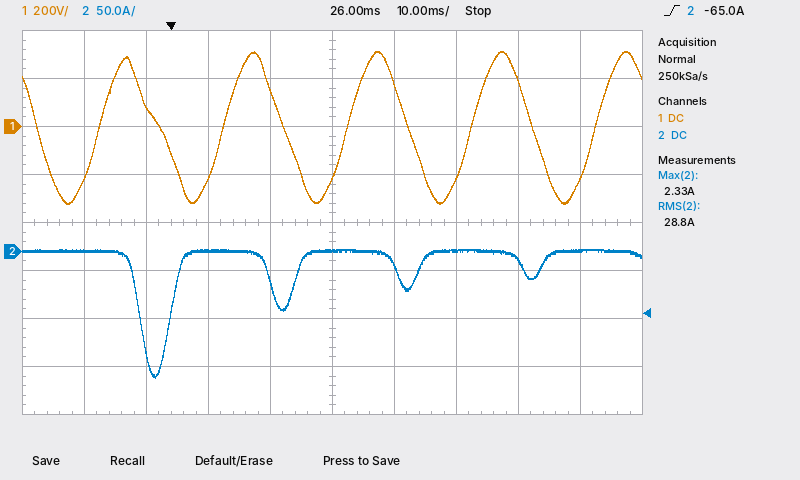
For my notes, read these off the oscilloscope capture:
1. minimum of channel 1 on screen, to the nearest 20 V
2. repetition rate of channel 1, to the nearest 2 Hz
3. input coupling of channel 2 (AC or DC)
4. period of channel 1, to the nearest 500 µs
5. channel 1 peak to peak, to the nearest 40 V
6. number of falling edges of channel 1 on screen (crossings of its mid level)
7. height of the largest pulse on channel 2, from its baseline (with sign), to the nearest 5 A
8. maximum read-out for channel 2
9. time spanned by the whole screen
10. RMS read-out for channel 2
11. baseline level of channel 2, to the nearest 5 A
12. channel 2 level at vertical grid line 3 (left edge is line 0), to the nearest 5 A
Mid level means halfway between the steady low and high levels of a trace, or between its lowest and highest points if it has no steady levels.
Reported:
-320 V
50 Hz
DC
20.0 ms
640 V
5
-130 A
2.33 A
100 ms
28.8 A
0 A
0 A
